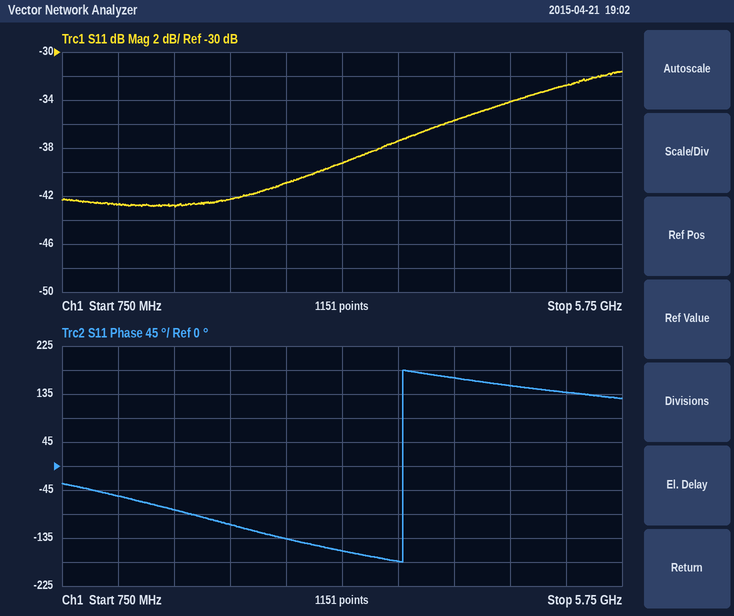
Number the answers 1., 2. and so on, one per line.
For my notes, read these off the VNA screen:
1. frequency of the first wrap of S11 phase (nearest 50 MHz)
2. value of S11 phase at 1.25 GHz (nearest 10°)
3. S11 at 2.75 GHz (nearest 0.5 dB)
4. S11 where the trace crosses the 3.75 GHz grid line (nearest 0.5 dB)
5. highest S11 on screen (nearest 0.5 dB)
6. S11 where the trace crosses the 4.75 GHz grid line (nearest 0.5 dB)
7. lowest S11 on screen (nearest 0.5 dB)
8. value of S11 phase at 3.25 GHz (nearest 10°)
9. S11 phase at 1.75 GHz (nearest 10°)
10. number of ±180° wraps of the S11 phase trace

1. 3.80 GHz
2. -60°
3. -41.0 dB
4. -37.5 dB
5. -31.5 dB
6. -34.0 dB
7. -43.0 dB
8. -160°
9. -80°
10. 1
